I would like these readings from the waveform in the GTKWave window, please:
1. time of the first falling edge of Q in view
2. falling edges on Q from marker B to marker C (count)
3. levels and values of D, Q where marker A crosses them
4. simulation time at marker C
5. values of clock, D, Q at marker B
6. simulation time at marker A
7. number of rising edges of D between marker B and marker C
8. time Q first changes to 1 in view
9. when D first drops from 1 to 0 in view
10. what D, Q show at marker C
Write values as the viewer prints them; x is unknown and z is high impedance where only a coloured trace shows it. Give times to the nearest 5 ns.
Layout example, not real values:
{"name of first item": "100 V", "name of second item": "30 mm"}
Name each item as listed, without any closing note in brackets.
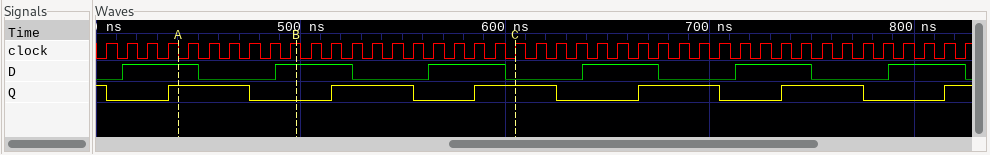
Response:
{"time of the first falling edge of Q in view": "405 ns", "falling edges on Q from marker B to marker C": "1", "levels and values of D, Q where marker A crosses them": "D=1, Q=1", "simulation time at marker C": "605 ns", "values of clock, D, Q at marker B": "clock=1, D=1, Q=0", "simulation time at marker A": "440 ns", "number of rising edges of D between marker B and marker C": "1", "time Q first changes to 1 in view": "435 ns", "when D first drops from 1 to 0 in view": "450 ns", "what D, Q show at marker C": "D=0, Q=1"}
